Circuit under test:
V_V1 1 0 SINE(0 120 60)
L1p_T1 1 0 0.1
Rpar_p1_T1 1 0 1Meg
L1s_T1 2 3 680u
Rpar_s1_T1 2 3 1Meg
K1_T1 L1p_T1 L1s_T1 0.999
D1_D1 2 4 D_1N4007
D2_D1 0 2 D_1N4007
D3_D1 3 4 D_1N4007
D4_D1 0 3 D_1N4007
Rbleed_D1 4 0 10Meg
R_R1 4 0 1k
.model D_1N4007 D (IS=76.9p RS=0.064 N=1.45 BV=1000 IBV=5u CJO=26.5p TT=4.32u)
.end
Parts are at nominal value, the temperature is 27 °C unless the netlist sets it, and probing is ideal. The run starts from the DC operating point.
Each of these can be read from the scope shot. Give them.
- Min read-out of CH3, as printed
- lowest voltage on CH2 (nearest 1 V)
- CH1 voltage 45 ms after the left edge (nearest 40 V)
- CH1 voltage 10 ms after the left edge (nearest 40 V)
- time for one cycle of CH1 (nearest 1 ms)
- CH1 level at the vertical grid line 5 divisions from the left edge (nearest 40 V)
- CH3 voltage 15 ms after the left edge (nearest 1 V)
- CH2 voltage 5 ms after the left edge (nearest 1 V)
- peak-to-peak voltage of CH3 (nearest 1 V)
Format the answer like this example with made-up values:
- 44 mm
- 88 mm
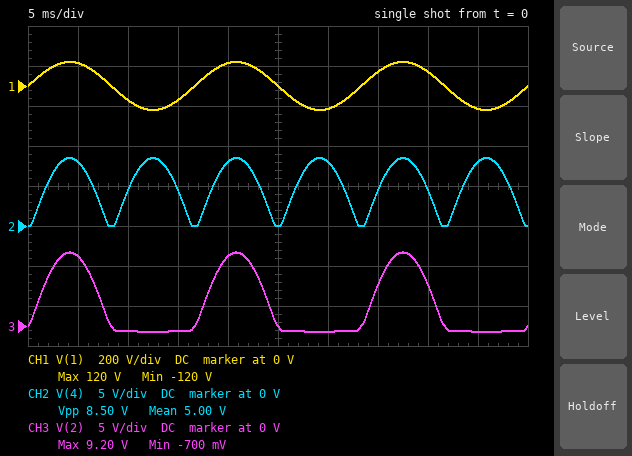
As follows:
- -700 mV
- 0 V
- -120 V
- -80 V
- 17 ms
- 0 V
- -1 V
- 8 V
- 10 V
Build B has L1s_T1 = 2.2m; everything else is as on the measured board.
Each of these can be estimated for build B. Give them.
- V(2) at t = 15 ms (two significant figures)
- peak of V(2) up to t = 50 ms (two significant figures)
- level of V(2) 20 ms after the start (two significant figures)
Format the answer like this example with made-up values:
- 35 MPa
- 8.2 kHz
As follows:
- -700 mV
- 17 V
- 16 V
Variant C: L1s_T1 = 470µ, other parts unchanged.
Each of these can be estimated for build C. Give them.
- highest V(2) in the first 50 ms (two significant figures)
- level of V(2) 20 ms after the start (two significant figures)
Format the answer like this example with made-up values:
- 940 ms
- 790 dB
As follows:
- 7.5 V
- 7.1 V
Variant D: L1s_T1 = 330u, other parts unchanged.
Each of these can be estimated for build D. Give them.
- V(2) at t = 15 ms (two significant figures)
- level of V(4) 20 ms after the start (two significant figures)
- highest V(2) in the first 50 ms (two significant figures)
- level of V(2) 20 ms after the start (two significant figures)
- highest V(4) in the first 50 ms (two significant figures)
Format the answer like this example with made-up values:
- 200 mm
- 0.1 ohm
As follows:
- -650 mV
- 5.2 V
- 6.2 V
- 5.9 V
- 5.5 V
